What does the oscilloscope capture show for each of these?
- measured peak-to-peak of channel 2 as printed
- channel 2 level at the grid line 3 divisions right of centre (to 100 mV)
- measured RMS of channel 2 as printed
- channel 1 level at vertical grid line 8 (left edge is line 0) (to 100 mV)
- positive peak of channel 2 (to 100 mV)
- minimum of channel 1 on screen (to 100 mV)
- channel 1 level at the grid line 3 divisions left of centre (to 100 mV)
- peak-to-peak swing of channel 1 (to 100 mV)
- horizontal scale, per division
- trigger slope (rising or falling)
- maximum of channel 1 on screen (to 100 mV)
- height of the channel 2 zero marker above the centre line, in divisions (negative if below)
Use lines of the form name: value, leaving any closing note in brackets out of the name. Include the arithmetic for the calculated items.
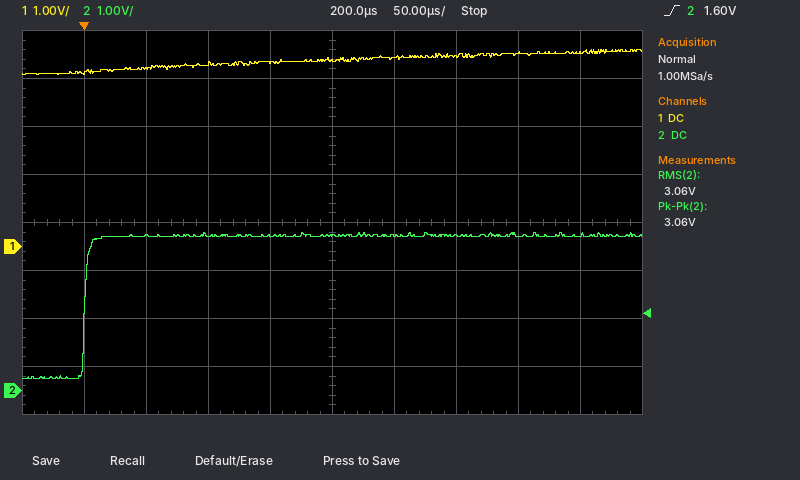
measured peak-to-peak of channel 2 as printed: 3.06 V
channel 2 level at the grid line 3 divisions right of centre: 3.2 V
measured RMS of channel 2 as printed: 3.06 V
channel 1 level at vertical grid line 8 (left edge is line 0): 4.0 V
positive peak of channel 2: 3.3 V
minimum of channel 1 on screen: 3.6 V
channel 1 level at the grid line 3 divisions left of centre: 3.7 V
peak-to-peak swing of channel 1: 4.1 V − (3.6 V) = 500 mV
horizontal scale, per division: 50 µs
trigger slope: rising
maximum of channel 1 on screen: 4.1 V
height of the channel 2 zero marker above the centre line, in divisions: -3.5 div
